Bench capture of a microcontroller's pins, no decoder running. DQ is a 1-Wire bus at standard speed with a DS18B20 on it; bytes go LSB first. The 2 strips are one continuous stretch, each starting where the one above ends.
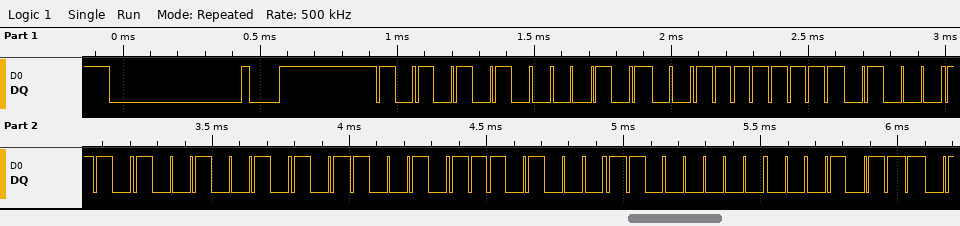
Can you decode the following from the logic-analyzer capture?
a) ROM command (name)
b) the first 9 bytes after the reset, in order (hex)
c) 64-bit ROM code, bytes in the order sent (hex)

Match ROM
55 28 FF 62 49 4D 17 03 E8
28 FF 62 49 4D 17 03 E8
